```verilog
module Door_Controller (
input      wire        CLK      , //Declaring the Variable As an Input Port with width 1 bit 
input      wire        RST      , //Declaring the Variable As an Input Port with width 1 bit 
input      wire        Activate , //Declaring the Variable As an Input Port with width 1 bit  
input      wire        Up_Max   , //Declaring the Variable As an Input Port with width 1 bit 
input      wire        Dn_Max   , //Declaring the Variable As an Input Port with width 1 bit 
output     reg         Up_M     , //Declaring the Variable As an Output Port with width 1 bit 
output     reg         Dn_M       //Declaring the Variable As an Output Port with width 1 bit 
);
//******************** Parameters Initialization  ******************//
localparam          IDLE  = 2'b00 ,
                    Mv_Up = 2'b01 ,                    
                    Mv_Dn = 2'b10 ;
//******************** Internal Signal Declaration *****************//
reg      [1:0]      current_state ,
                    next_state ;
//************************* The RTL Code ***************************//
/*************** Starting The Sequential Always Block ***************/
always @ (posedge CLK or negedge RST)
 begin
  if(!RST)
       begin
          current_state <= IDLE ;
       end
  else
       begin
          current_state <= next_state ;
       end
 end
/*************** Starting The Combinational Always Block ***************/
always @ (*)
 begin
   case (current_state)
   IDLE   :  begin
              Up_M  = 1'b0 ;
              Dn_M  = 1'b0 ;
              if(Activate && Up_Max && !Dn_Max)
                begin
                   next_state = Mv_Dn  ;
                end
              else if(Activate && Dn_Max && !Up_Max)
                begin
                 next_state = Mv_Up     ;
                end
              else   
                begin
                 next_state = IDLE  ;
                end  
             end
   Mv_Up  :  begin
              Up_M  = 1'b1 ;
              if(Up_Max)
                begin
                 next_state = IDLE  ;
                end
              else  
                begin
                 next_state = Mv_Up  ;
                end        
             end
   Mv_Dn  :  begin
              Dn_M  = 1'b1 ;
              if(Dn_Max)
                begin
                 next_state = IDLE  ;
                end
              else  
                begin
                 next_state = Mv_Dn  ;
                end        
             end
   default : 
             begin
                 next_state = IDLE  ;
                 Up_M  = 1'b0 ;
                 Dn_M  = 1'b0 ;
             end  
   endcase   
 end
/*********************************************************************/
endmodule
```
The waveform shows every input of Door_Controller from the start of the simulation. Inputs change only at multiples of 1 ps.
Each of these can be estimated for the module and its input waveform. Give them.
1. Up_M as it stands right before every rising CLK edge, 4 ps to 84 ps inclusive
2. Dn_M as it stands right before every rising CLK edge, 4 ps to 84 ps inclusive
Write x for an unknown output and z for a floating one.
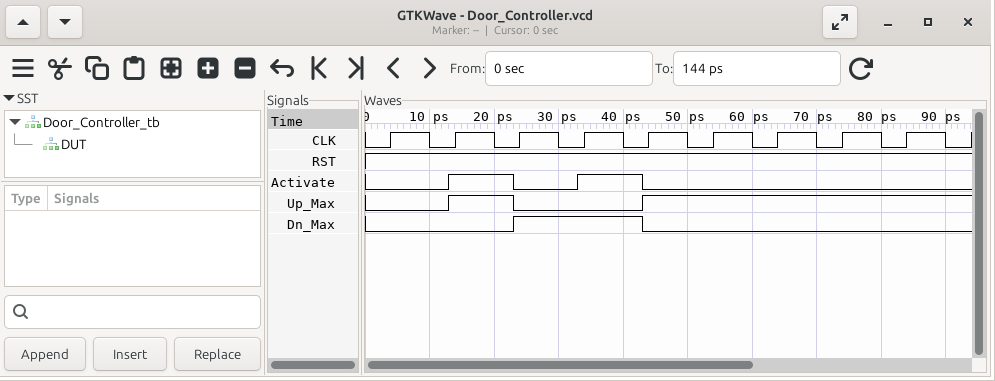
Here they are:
0 0 0 0 1 0 0 0 0
0 0 1 0 0 0 0 0 0
